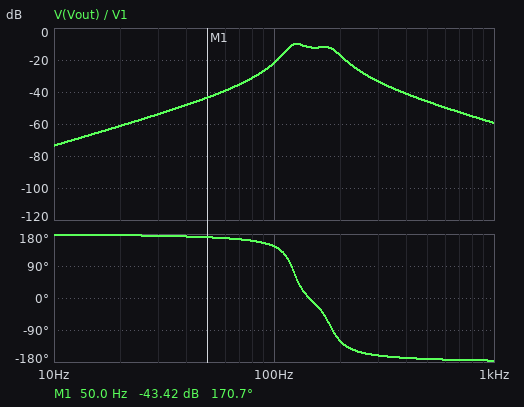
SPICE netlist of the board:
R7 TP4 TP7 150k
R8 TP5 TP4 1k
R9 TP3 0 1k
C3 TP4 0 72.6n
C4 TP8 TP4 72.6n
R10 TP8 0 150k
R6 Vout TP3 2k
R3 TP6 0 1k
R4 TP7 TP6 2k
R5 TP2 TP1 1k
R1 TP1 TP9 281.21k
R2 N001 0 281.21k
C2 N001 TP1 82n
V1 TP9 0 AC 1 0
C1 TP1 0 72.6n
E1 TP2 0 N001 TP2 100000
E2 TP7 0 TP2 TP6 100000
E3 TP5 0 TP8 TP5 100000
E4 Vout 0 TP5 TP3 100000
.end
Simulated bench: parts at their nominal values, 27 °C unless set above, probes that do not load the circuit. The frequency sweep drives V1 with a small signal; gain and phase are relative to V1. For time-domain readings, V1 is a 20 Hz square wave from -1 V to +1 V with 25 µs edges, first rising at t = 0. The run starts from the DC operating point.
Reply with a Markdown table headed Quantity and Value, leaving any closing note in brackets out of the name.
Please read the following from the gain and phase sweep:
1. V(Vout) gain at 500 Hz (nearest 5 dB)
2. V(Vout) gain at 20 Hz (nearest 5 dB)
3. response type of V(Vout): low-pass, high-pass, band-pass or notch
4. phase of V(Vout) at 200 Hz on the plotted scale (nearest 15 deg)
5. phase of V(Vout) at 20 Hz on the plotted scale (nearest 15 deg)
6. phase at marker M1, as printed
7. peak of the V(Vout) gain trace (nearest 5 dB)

| Quantity | Value |
|---|---|
| V(Vout) gain at 500 Hz | -45 dB |
| V(Vout) gain at 20 Hz | -60 dB |
| response type of V(Vout): low-pass, high-pass, band-pass or notch | band-pass |
| phase of V(Vout) at 200 Hz on the plotted scale | -120 deg |
| phase of V(Vout) at 20 Hz on the plotted scale | 180 deg |
| phase at marker M1, as printed | 170.7 deg |
| peak of the V(Vout) gain trace | -10 dB |
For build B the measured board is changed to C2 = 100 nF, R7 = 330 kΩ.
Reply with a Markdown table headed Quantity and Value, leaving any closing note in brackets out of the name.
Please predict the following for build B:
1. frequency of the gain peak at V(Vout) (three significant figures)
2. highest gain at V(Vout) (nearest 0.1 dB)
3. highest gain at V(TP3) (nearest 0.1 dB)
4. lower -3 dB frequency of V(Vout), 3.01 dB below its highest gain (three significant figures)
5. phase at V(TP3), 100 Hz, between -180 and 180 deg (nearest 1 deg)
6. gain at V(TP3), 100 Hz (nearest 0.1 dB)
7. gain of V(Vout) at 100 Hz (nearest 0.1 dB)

| Quantity | Value |
|---|---|
| frequency of the gain peak at V(Vout) | 114 Hz |
| highest gain at V(Vout) | -18.1 dB |
| highest gain at V(TP3) | -27.6 dB |
| lower -3 dB frequency of V(Vout), 3.01 dB below its highest gain | 105 Hz |
| phase at V(TP3), 100 Hz, between -180 and 180 deg | 130 deg |
| gain at V(TP3), 100 Hz | -33.4 dB |
| gain of V(Vout) at 100 Hz | -23.9 dB |
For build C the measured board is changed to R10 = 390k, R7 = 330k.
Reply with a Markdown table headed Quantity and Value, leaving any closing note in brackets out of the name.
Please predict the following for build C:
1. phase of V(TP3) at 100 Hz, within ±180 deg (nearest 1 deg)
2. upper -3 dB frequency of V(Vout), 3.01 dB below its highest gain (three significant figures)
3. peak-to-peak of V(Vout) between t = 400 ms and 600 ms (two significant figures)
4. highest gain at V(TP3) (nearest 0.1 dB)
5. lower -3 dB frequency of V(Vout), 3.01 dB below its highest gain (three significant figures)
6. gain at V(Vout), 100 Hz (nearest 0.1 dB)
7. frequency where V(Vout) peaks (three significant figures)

| Quantity | Value |
|---|---|
| phase of V(TP3) at 100 Hz, within ±180 deg | 119 deg |
| upper -3 dB frequency of V(Vout), 3.01 dB below its highest gain | 126 Hz |
| peak-to-peak of V(Vout) between t = 400 ms and 600 ms | 200 mV |
| highest gain at V(TP3) | -10.9 dB |
| lower -3 dB frequency of V(Vout), 3.01 dB below its highest gain | 108 Hz |
| gain at V(Vout), 100 Hz | -11.1 dB |
| frequency where V(Vout) peaks | 116 Hz |
